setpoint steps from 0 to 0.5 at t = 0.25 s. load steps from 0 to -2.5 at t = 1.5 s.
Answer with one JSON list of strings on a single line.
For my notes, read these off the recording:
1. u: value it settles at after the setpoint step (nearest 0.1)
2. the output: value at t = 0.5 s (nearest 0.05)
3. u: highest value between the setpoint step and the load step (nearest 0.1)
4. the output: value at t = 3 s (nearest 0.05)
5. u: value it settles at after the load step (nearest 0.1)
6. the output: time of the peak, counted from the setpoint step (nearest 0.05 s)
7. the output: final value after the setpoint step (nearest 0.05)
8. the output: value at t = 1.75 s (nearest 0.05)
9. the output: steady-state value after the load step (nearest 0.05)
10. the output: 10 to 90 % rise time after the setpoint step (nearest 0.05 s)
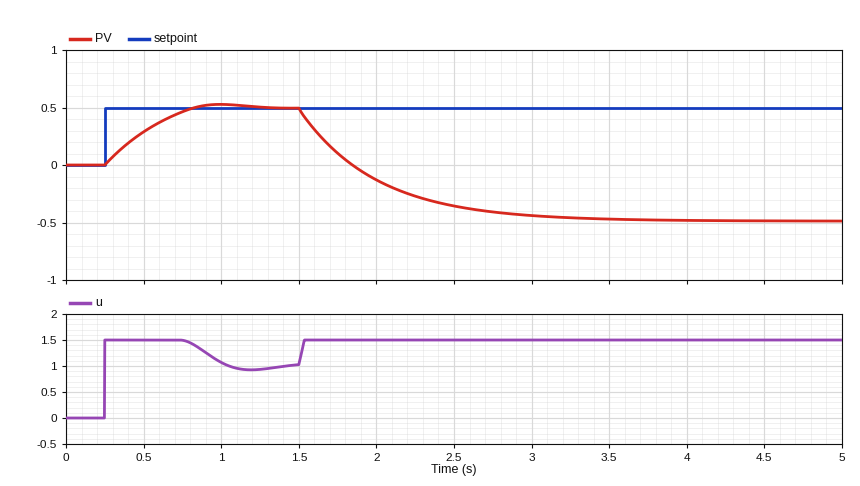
["1.0", "0.30", "1.5", "-0.45", "1.5", "0.75 s", "0.50", "0.10", "-0.50", "0.45 s"]
